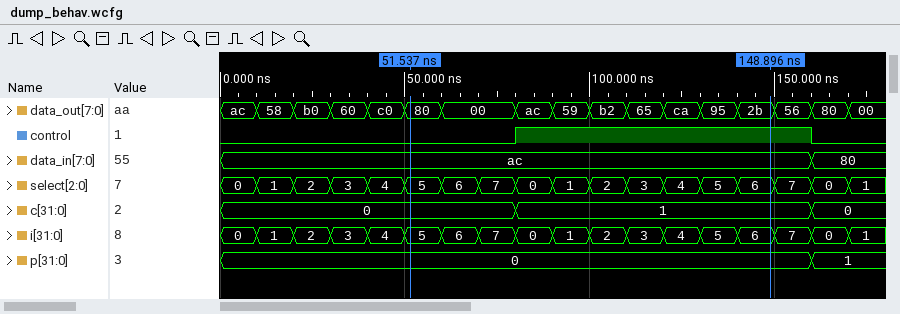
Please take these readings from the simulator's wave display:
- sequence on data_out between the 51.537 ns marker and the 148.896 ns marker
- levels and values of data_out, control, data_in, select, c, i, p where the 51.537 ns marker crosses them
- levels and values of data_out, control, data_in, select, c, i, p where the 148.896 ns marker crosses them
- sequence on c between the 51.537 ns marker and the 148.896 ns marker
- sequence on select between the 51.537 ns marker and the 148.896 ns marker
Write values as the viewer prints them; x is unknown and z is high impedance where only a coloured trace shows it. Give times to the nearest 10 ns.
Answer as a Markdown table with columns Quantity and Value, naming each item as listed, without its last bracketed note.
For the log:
| Quantity | Value |
|---|---|
| sequence on data_out between the 51.537 ns marker and the 148.896 ns marker | 80, 00, ac, 59, b2, 65, ca, 95, 2b |
| levels and values of data_out, control, data_in, select, c, i, p where the 51.537 ns marker crosses them | data_out=80, control=0, data_in=ac, select=5, c=0, i=5, p=0 |
| levels and values of data_out, control, data_in, select, c, i, p where the 148.896 ns marker crosses them | data_out=2b, control=1, data_in=ac, select=6, c=1, i=6, p=0 |
| sequence on c between the 51.537 ns marker and the 148.896 ns marker | 0, 1 |
| sequence on select between the 51.537 ns marker and the 148.896 ns marker | 5, 6, 7, 0, 1, 2, 3, 4, 5, 6 |
